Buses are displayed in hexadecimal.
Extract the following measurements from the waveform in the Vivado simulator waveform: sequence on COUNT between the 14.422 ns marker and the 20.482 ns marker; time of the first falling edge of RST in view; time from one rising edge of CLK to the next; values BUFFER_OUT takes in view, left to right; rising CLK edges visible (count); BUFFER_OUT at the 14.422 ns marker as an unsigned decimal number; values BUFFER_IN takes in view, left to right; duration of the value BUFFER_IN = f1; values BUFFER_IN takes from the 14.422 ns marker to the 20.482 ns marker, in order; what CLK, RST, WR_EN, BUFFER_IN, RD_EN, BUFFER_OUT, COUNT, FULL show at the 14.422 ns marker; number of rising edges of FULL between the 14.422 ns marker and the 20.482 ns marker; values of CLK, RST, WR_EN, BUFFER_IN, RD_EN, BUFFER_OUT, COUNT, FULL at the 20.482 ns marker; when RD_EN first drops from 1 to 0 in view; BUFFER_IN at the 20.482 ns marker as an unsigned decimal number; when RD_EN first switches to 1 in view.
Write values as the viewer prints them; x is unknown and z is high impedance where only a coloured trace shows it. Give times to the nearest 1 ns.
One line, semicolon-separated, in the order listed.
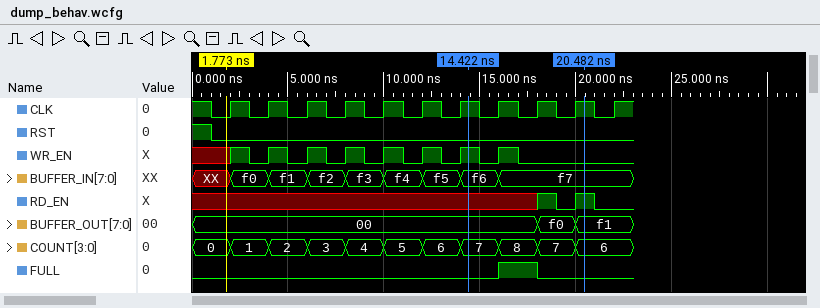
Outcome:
7, 8, 7, 6; 1 ns; 2 ns; 00, f0, f1; 11; 0; XX, f0, f1, f2, f3, f4, f5, f6, f7; 2 ns; f6, f7; CLK=1, RST=0, WR_EN=1, BUFFER_IN=f6, RD_EN=x, BUFFER_OUT=00, COUNT=7, FULL=0; 1; CLK=1, RST=0, WR_EN=0, BUFFER_IN=f7, RD_EN=1, BUFFER_OUT=f1, COUNT=6, FULL=0; 19 ns; 247; 18 ns
